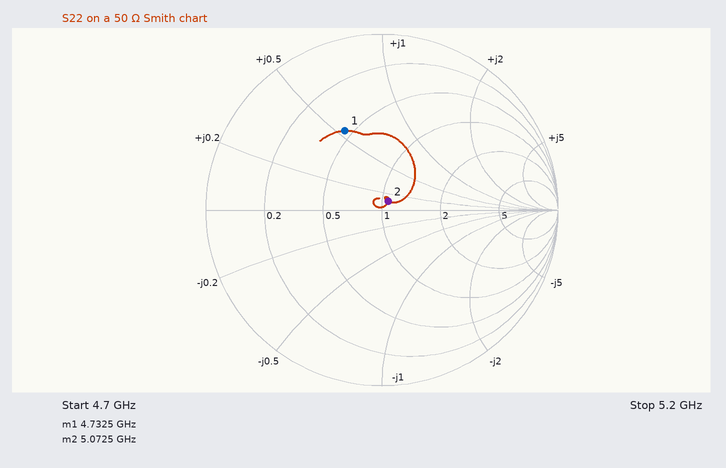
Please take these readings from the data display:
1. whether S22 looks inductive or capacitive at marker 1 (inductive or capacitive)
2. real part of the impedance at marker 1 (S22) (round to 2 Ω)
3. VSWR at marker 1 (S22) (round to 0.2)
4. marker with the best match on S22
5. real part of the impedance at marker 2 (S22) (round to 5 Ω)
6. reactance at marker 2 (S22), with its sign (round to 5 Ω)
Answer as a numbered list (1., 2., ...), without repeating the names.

1. inductive
2. 22 Ω
3. 3.0
4. marker 2
5. 55 Ω
6. +5 Ω
